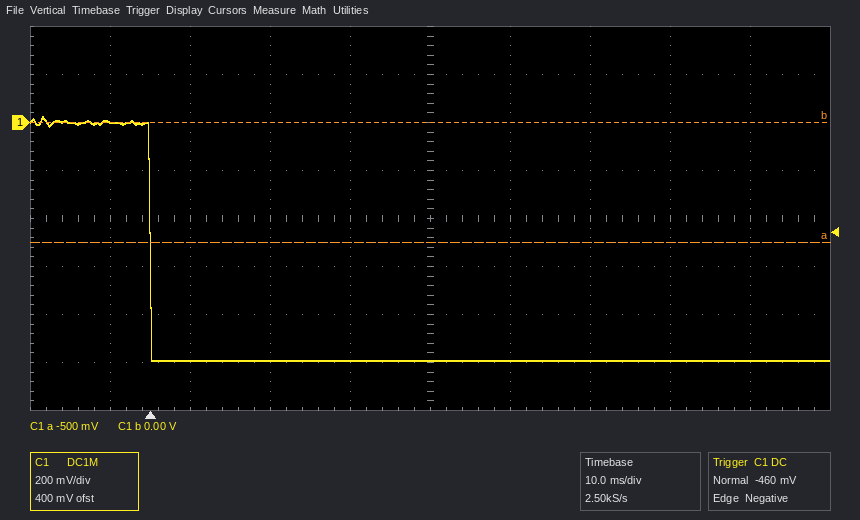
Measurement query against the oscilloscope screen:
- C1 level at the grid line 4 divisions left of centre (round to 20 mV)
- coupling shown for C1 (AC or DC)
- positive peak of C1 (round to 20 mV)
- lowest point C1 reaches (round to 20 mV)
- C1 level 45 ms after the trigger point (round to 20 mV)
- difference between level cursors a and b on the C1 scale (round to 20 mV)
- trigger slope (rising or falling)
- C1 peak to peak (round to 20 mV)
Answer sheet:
0 mV
DC
20 mV
-1.00 V
-1.00 V
500 mV
falling
1.02 V
